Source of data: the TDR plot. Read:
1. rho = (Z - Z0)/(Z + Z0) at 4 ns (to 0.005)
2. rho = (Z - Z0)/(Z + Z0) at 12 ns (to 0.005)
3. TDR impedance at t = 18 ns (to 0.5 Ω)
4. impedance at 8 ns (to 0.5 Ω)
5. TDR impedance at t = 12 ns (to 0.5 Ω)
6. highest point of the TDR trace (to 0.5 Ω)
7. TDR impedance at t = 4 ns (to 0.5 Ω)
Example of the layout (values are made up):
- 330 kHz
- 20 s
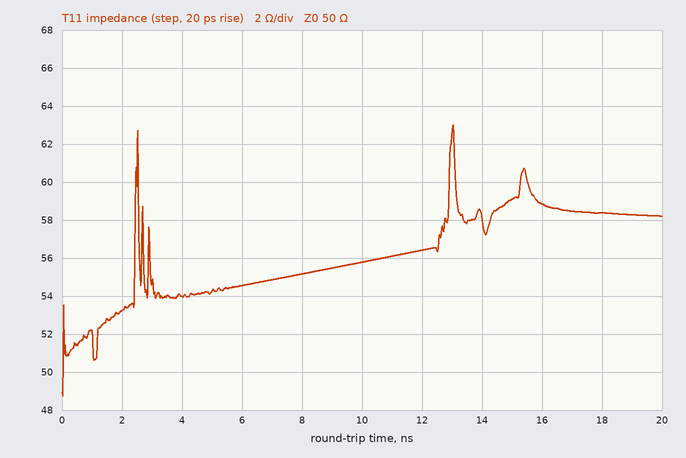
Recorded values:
- +0.040
- +0.060
- 58.5 Ω
- 55.0 Ω
- 56.5 Ω
- 63.0 Ω
- 54.0 Ω
